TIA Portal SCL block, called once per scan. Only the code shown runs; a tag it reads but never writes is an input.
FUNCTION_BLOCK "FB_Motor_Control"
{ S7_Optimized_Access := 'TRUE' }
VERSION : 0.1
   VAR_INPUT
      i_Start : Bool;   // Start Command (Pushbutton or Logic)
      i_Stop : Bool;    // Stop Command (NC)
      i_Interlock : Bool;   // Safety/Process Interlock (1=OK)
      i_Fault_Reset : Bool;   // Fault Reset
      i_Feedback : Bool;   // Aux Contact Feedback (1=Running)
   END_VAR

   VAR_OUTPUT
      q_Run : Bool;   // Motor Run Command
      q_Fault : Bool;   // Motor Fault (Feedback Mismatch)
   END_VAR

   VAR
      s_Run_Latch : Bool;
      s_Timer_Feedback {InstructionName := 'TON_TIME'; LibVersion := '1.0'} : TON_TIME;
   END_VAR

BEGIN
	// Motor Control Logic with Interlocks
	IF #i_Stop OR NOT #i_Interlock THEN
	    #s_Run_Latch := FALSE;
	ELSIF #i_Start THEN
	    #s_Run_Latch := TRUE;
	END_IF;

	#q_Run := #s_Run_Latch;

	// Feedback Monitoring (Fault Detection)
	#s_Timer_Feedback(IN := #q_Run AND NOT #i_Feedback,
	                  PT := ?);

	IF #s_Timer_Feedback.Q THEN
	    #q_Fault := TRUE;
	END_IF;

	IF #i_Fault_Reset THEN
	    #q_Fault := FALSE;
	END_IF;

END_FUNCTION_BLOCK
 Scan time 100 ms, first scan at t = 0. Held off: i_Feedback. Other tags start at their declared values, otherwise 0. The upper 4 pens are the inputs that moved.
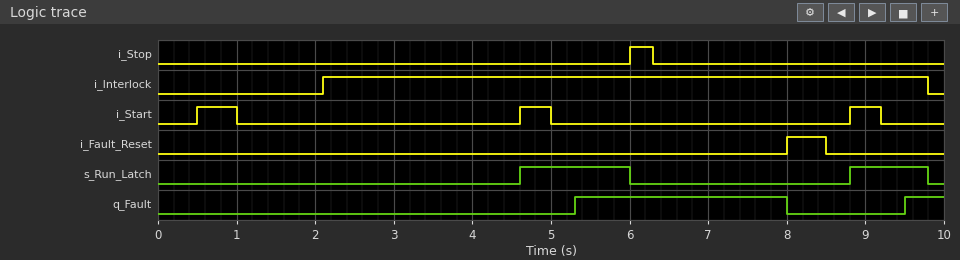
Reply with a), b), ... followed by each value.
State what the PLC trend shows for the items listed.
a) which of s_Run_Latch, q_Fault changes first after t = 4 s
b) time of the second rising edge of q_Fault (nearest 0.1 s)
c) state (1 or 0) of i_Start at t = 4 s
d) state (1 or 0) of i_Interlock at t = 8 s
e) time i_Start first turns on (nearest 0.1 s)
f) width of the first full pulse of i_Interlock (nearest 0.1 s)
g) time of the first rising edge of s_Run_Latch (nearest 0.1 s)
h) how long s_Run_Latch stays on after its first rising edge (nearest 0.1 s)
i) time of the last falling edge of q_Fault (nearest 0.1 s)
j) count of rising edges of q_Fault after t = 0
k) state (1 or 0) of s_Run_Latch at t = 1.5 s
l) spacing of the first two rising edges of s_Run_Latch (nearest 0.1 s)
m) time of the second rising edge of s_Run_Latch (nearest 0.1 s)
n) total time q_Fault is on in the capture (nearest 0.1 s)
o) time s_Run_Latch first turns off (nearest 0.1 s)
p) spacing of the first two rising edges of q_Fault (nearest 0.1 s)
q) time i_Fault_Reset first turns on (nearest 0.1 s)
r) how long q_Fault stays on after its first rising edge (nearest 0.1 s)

a) s_Run_Latch
b) 9.5 s
c) 0
d) 1
e) 0.5 s
f) 7.7 s
g) 4.6 s
h) 1.4 s
i) 8.0 s
j) 2
k) 0
l) 4.2 s
m) 8.8 s
n) 3.2 s
o) 6.0 s
p) 4.2 s
q) 8.0 s
r) 2.7 s
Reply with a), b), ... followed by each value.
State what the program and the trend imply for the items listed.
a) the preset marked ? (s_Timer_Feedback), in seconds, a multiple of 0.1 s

a) 0.7 s
